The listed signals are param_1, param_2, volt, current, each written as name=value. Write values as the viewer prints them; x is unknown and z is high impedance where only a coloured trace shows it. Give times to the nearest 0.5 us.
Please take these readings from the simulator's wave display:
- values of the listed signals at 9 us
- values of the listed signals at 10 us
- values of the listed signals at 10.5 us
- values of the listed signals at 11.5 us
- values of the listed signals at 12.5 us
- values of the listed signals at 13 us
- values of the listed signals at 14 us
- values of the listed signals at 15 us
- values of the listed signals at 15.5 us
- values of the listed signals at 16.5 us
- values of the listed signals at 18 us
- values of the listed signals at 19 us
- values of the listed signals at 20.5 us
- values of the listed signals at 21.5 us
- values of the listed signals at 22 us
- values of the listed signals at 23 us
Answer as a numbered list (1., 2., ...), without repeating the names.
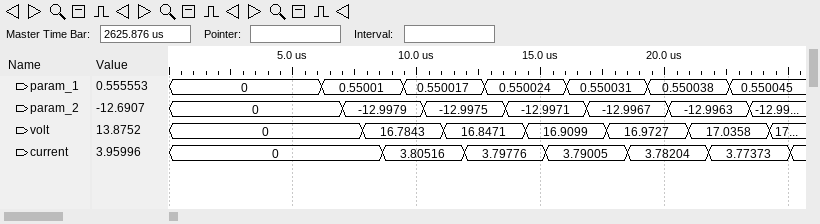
1. param_1=0.55001, param_2=-12.9979, volt=16.7843, current=3.80516
2. param_1=0.550017, param_2=-12.9979, volt=16.7843, current=3.80516
3. param_1=0.550017, param_2=-12.9975, volt=16.7843, current=3.80516
4. param_1=0.550017, param_2=-12.9975, volt=16.8471, current=3.80516
5. param_1=0.550017, param_2=-12.9975, volt=16.8471, current=3.79776
6. param_1=0.550024, param_2=-12.9975, volt=16.8471, current=3.79776
7. param_1=0.550024, param_2=-12.9971, volt=16.8471, current=3.79776
8. param_1=0.550024, param_2=-12.9971, volt=16.9099, current=3.79776
9. param_1=0.550024, param_2=-12.9971, volt=16.9099, current=3.79005
10. param_1=0.550031, param_2=-12.9971, volt=16.9099, current=3.79005
11. param_1=0.550031, param_2=-12.9967, volt=16.9727, current=3.79005
12. param_1=0.550031, param_2=-12.9967, volt=16.9727, current=3.78204
13. param_1=0.550038, param_2=-12.9963, volt=16.9727, current=3.78204
14. param_1=0.550038, param_2=-12.9963, volt=17.0358, current=3.78204
15. param_1=0.550038, param_2=-12.9963, volt=17.0358, current=3.77373
16. param_1=0.550045, param_2=-12.9963, volt=17.0358, current=3.77373
